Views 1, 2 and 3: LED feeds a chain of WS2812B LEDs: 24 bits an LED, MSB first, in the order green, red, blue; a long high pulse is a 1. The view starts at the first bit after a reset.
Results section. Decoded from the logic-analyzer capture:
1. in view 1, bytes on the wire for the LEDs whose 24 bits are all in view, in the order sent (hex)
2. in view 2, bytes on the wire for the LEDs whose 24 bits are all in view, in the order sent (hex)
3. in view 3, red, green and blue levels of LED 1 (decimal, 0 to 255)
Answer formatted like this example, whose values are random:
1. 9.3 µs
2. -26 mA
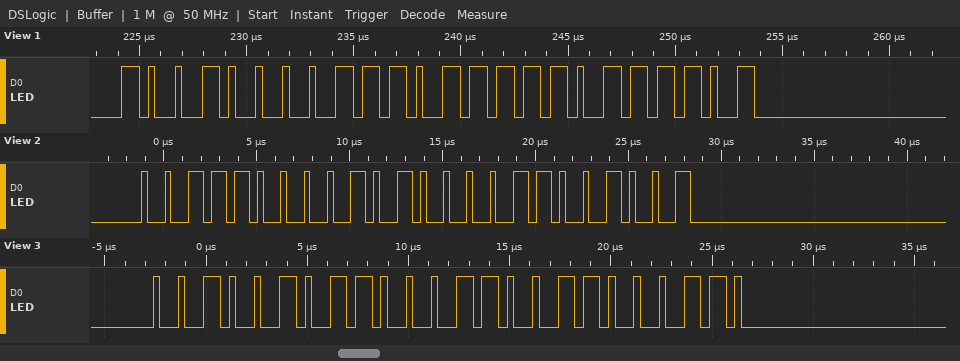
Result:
1. 90 EF BD
2. 38 50 C9
3. 140, 37, 198
